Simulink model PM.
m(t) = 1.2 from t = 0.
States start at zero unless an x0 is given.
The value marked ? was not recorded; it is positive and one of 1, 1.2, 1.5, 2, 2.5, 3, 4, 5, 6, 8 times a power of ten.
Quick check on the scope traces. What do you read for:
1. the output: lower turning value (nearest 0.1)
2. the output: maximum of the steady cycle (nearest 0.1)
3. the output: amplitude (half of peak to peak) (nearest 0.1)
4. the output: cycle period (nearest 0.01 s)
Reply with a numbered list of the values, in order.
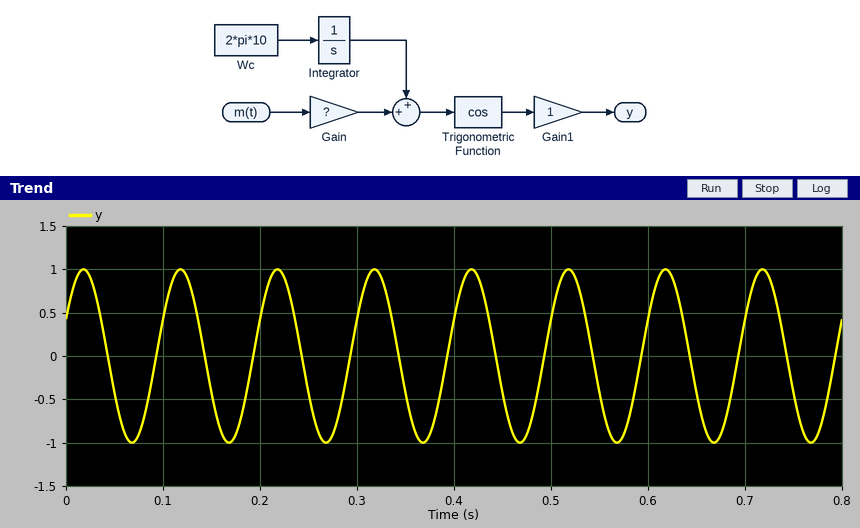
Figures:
1. -1.0
2. 1.0
3. 1.0
4. 0.10 s
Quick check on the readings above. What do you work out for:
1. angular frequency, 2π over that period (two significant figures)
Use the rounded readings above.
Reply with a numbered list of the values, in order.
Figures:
1. 63 rad/s
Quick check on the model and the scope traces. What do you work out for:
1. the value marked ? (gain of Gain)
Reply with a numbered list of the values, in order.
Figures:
1. 20
